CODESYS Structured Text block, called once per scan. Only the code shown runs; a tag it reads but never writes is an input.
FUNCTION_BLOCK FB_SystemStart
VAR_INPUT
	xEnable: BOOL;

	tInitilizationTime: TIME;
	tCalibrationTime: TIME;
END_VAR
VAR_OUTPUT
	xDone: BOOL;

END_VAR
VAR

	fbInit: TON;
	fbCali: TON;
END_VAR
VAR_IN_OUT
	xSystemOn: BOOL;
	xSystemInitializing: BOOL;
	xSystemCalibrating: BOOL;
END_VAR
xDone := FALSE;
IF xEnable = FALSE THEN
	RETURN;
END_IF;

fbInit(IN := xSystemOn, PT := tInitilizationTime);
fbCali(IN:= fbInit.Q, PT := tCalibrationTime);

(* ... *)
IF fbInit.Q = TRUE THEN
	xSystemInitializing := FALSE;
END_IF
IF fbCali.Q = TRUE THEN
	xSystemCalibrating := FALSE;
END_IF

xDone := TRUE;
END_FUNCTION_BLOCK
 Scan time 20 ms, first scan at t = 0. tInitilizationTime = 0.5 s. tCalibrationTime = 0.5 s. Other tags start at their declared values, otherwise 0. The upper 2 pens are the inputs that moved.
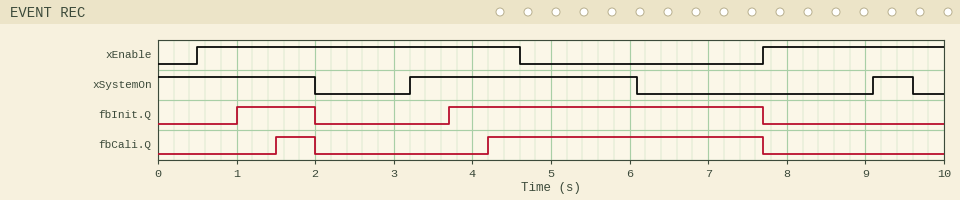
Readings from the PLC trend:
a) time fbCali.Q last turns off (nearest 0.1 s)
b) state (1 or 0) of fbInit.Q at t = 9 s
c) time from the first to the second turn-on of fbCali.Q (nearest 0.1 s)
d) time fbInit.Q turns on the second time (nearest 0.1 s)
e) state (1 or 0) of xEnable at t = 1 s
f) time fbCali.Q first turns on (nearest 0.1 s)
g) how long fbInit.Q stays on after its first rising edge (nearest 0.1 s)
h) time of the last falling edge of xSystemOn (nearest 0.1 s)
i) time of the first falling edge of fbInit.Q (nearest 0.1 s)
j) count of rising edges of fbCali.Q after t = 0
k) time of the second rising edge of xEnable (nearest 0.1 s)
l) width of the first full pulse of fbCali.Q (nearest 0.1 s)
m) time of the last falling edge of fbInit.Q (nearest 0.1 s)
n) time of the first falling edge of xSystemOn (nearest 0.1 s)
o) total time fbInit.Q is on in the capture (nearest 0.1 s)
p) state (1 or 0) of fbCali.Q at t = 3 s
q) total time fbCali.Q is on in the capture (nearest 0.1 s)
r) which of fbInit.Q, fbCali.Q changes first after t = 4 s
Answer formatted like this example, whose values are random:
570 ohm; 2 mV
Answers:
7.7 s; 0; 2.7 s; 3.7 s; 1; 1.5 s; 1.0 s; 9.6 s; 2.0 s; 2; 7.7 s; 0.5 s; 7.7 s; 2.0 s; 5.0 s; 0; 4.0 s; fbCali.Q
